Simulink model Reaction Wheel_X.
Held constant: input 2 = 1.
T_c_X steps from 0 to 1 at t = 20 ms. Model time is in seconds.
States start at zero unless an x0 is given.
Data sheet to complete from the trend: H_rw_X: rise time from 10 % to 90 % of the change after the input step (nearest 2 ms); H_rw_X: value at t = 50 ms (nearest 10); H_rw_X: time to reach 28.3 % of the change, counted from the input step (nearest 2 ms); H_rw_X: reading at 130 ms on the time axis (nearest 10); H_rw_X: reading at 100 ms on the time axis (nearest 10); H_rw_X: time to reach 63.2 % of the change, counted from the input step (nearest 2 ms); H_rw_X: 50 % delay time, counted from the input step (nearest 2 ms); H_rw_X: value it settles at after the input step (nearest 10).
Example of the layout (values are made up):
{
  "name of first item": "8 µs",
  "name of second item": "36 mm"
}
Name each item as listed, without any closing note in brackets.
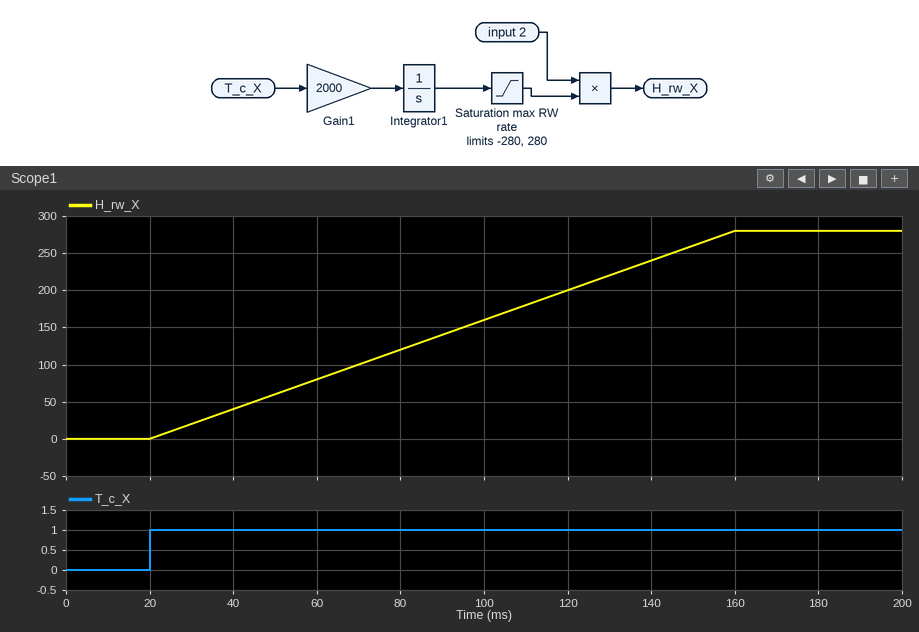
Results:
{
  "H_rw_X: rise time from 10 % to 90 % of the change after the input step": "112 ms",
  "H_rw_X: value at t = 50 ms": "60",
  "H_rw_X: time to reach 28.3 % of the change, counted from the input step": "40 ms",
  "H_rw_X: reading at 130 ms on the time axis": "220",
  "H_rw_X: reading at 100 ms on the time axis": "160",
  "H_rw_X: time to reach 63.2 % of the change, counted from the input step": "88 ms",
  "H_rw_X: 50 % delay time, counted from the input step": "70 ms",
  "H_rw_X: value it settles at after the input step": "280"
}
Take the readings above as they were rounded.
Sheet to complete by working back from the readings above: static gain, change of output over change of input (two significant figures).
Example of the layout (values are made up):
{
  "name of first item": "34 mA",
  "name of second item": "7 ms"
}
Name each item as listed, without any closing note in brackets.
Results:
{
  "static gain, change of output over change of input": "280"
}
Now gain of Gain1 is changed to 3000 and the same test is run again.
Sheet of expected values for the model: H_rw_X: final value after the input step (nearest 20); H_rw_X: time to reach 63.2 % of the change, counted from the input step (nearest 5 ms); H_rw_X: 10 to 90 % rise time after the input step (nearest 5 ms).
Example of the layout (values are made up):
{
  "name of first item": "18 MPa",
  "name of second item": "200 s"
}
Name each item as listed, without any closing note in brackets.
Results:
{
  "H_rw_X: final value after the input step": "280",
  "H_rw_X: time to reach 63.2 % of the change, counted from the input step": "60 ms",
  "H_rw_X: 10 to 90 % rise time after the input step": "75 ms"
}
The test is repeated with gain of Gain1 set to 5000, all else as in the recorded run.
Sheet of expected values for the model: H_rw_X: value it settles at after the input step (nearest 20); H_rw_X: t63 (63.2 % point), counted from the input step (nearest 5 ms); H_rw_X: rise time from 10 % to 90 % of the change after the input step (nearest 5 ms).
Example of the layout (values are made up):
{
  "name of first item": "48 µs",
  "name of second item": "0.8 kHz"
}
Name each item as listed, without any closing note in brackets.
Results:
{
  "H_rw_X: value it settles at after the input step": "280",
  "H_rw_X: t63 (63.2 % point), counted from the input step": "35 ms",
  "H_rw_X: rise time from 10 % to 90 % of the change after the input step": "45 ms"
}
